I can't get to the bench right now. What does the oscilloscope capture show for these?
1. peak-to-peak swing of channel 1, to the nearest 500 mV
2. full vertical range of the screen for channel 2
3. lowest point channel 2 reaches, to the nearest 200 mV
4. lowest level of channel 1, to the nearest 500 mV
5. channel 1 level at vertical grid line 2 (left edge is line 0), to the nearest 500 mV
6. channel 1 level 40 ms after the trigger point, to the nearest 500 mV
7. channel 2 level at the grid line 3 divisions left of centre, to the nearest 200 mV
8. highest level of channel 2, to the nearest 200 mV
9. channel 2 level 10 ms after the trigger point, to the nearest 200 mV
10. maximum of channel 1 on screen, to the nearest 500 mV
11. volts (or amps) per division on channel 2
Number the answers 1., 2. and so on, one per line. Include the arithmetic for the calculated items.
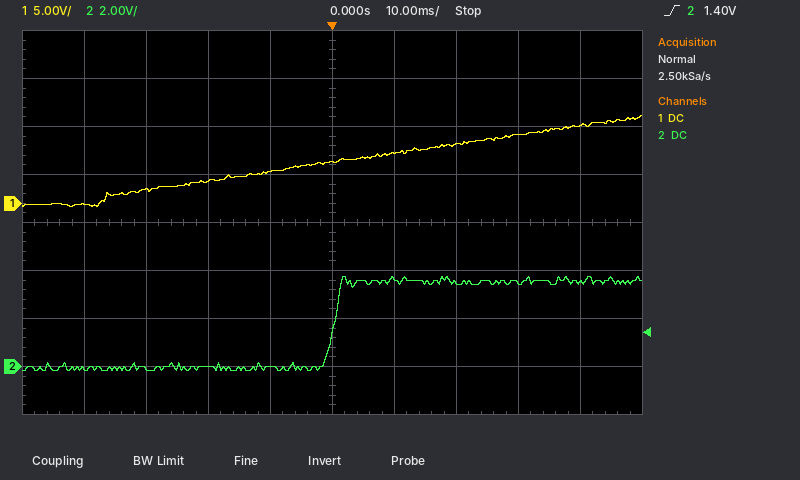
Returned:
1. 9.0 V − (-500 mV) = 9.5 V
2. 16 V
3. -200 mV
4. -500 mV
5. 1.5 V
6. 8.0 V
7. 0.0 V
8. 3.8 V
9. 3.6 V
10. 9.0 V
11. 2 V
